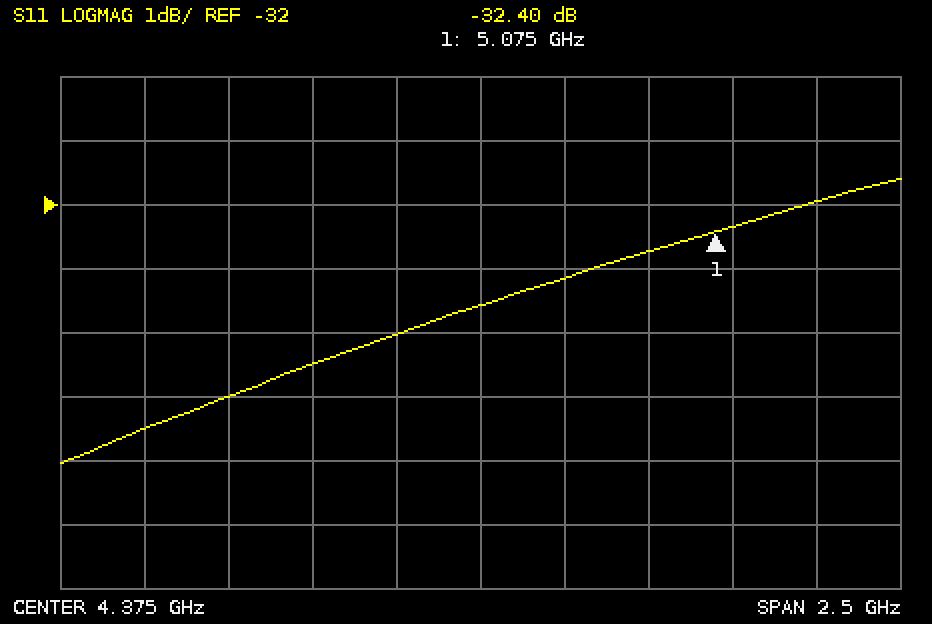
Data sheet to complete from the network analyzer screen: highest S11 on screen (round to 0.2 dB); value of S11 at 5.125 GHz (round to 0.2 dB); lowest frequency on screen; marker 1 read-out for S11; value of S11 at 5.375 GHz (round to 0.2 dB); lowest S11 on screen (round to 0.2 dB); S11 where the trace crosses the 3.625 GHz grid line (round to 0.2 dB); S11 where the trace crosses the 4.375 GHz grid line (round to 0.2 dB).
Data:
-31.6 dB
-32.4 dB
3.125 GHz
-32.40 dB
-32.0 dB
-36.0 dB
-35.0 dB
-33.6 dB
